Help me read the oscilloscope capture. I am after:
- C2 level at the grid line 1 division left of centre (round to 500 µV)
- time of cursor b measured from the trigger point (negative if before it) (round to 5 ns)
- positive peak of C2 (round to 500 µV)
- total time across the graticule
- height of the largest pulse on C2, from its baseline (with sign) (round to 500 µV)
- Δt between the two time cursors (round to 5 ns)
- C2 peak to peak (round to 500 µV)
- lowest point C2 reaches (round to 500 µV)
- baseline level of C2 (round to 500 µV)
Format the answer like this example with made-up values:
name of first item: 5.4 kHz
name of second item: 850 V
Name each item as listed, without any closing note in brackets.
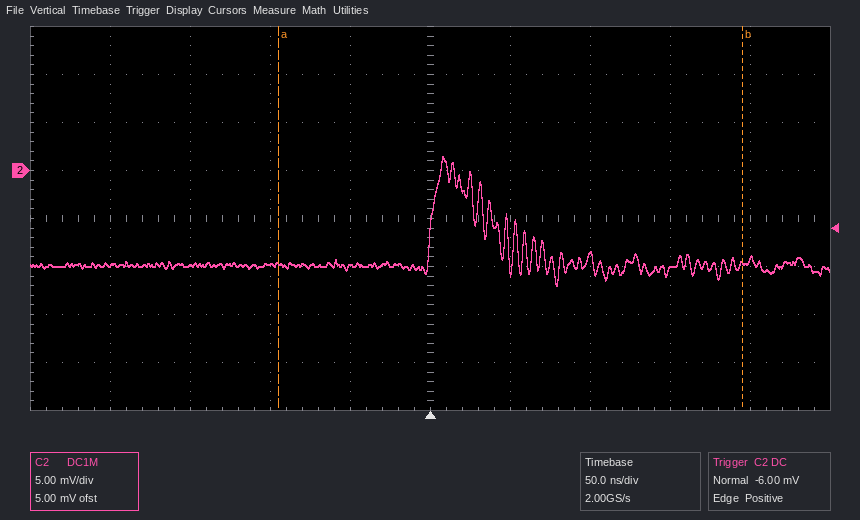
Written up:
C2 level at the grid line 1 division left of centre: -10.0 mV
time of cursor b measured from the trigger point (negative if before it): +195 ns
positive peak of C2: 1.5 mV
total time across the graticule: 500 ns
height of the largest pulse on C2, from its baseline (with sign): +11.5 mV
Δt between the two time cursors: 290 ns
C2 peak to peak: 13.5 mV
lowest point C2 reaches: -12.0 mV
baseline level of C2: -10.0 mV
